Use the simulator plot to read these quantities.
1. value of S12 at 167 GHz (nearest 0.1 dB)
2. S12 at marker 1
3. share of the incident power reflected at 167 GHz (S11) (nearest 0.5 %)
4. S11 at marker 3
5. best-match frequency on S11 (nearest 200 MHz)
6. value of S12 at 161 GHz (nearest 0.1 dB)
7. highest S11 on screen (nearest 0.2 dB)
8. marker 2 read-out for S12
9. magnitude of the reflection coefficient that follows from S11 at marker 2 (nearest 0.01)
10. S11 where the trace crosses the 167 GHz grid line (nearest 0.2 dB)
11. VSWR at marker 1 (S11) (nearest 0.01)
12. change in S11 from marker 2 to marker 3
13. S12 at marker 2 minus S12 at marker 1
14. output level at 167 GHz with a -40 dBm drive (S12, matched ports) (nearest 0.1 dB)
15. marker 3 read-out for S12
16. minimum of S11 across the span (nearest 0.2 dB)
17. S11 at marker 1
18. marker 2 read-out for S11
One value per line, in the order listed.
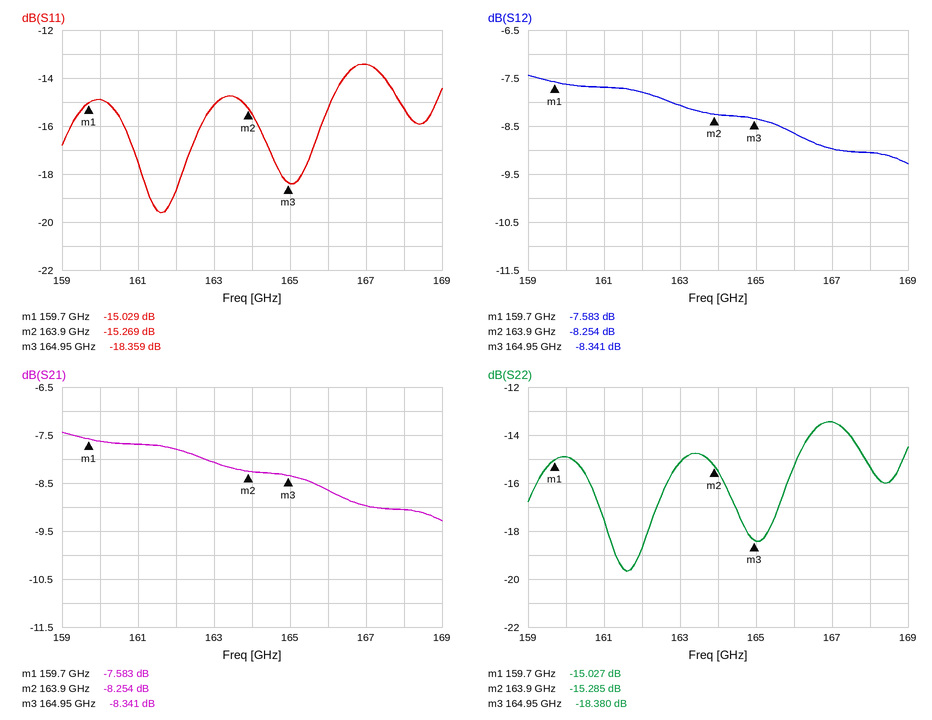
-9.0 dB
-7.583 dB
4.5 %
-18.359 dB
161.6 GHz
-7.7 dB
-13.4 dB
-8.254 dB
0.17
-13.4 dB
1.43
-3.090 dB
-0.671 dB
-49.0 dBm
-8.341 dB
-19.6 dB
-15.029 dB
-15.269 dB
